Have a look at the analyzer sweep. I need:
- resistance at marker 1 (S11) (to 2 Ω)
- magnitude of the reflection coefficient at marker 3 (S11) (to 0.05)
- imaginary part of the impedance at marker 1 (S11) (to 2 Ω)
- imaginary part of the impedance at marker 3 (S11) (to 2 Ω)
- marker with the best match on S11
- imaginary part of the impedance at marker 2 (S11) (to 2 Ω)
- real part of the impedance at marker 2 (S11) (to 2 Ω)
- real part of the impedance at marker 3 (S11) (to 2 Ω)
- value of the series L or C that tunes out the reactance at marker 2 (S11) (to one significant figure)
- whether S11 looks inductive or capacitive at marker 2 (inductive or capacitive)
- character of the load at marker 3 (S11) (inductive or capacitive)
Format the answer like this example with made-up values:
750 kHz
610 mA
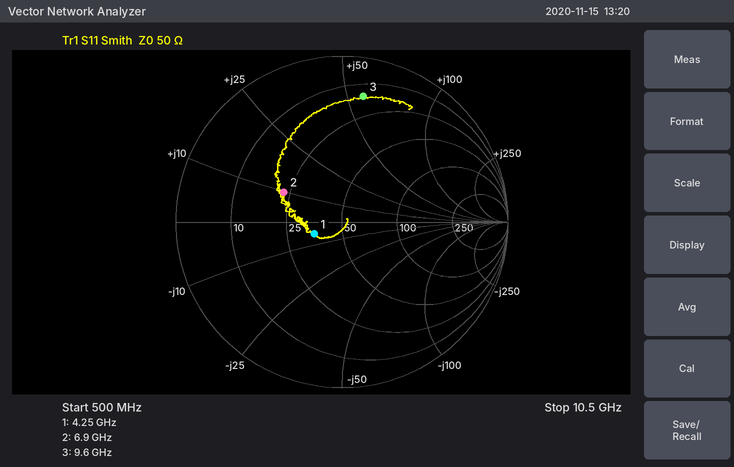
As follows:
36 Ω
0.75
-6 Ω
+56 Ω
marker 1
+10 Ω
22 Ω
16 Ω
2 pF
inductive
inductive
